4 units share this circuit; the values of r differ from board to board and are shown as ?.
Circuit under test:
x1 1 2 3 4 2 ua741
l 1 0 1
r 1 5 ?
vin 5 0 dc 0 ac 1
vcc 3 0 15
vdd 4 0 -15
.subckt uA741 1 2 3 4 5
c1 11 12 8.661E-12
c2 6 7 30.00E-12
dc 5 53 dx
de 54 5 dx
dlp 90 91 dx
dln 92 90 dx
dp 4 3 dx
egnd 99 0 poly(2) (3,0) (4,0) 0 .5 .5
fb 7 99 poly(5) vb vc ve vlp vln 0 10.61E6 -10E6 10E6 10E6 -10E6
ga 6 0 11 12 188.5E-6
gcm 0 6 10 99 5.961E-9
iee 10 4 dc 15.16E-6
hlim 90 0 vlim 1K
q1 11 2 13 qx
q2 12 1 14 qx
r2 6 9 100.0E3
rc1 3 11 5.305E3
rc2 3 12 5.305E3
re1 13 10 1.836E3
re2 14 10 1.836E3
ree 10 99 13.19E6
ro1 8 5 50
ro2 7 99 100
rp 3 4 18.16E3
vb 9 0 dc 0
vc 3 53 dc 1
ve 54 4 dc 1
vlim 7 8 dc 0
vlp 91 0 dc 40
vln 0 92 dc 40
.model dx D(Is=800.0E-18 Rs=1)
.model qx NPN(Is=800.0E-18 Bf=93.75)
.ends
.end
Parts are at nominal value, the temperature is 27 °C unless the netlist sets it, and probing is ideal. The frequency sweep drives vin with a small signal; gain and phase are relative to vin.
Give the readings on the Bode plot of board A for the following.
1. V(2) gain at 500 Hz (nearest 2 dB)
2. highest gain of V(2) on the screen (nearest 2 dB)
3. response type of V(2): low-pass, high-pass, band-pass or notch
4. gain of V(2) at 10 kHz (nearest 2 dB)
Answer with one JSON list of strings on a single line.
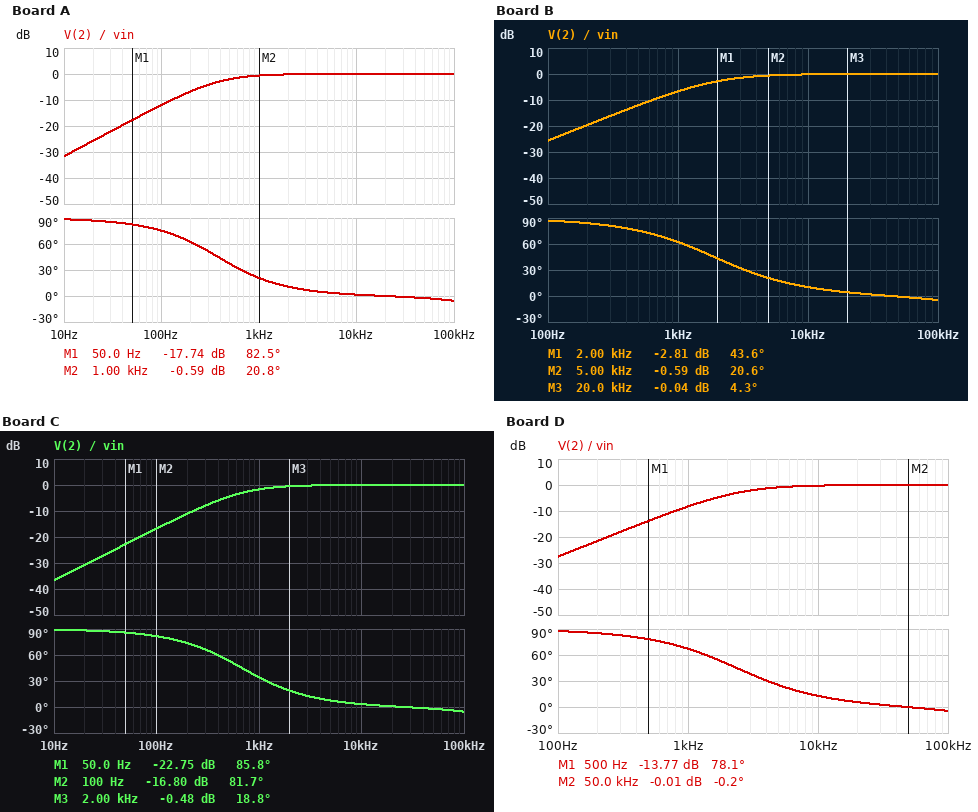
["-2 dB", "0 dB", "high-pass", "0 dB"]
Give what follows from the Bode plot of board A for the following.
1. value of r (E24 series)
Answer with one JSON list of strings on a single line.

["2.4 kΩ"]
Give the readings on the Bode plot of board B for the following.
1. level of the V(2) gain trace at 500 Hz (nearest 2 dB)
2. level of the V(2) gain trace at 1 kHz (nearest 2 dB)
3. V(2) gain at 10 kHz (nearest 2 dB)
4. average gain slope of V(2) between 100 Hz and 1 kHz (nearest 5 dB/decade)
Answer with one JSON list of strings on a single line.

["-12 dB", "-6 dB", "0 dB", "20 dB/decade"]
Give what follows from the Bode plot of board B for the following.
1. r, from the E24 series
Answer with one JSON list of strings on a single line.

["12 kΩ"]
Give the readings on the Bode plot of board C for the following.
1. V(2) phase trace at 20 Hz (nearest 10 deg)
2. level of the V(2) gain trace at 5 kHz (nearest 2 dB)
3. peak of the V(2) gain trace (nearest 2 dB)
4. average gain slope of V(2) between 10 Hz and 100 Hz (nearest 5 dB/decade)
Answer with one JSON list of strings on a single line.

["90 deg", "0 dB", "0 dB", "20 dB/decade"]
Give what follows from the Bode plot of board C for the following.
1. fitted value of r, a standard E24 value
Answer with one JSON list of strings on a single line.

["4.3 kΩ"]
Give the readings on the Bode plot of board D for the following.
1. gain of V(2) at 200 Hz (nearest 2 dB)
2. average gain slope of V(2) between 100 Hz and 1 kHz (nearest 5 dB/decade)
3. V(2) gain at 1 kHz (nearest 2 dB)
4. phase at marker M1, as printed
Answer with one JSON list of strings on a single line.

["-22 dB", "20 dB/decade", "-8 dB", "78.1 deg"]
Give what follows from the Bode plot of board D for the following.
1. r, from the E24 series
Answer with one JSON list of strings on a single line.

["15 kΩ"]
